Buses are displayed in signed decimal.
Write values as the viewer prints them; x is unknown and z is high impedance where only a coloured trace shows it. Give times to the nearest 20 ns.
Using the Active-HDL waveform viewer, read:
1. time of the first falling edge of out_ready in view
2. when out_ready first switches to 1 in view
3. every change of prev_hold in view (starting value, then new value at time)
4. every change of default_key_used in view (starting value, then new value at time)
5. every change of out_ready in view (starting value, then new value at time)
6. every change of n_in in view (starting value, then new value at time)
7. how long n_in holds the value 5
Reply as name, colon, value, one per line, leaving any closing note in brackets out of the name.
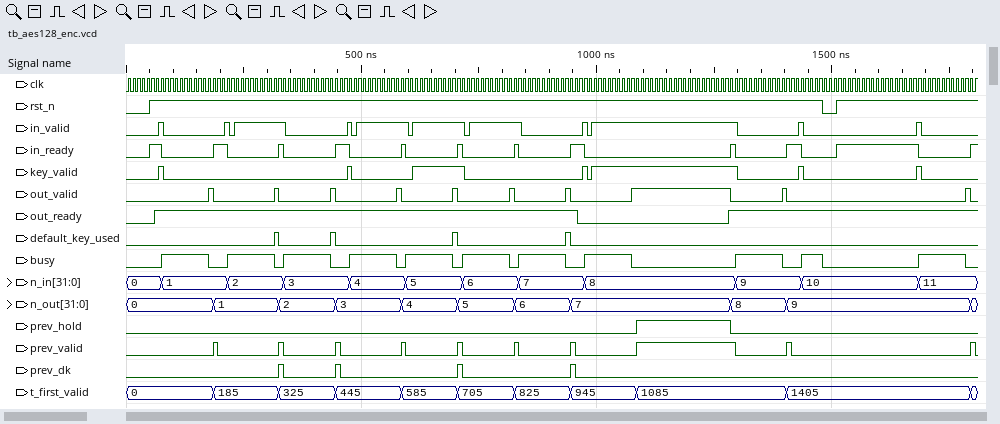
time of the first falling edge of out_ready in view: 960 ns
when out_ready first switches to 1 in view: 60 ns
every change of prev_hold in view: 0, 1 at 1080 ns, 0 at 1280 ns
every change of default_key_used in view: 0, 1 at 320 ns, 0 at 320 ns, 1 at 440 ns, 0 at 440 ns, 1 at 700 ns, 0 at 700 ns, 1 at 940 ns, 0 at 940 ns
every change of out_ready in view: 0, 1 at 60 ns, 0 at 960 ns, 1 at 1280 ns
every change of n_in in view: 0, 1 at 80 ns, 2 at 220 ns, 3 at 340 ns, 4 at 480 ns, 5 at 600 ns, 6 at 720 ns, 7 at 840 ns, 8 at 980 ns, 9 at 1300 ns, 10 at 1440 ns, 11 at 1680 ns
how long n_in holds the value 5: 120 ns
